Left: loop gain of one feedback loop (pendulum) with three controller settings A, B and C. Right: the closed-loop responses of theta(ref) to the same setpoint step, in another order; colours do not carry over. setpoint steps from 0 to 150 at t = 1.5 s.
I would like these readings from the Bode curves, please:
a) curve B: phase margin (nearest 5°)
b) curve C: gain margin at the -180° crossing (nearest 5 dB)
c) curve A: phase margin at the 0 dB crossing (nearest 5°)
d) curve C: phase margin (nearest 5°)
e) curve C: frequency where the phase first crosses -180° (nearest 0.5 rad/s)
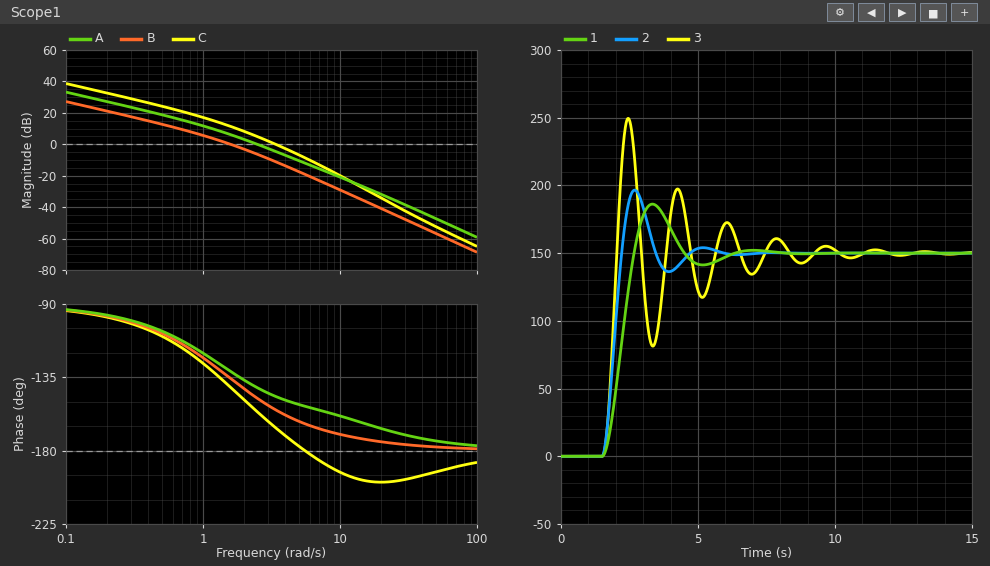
45°
10 dB
40°
15°
5.5 rad/s
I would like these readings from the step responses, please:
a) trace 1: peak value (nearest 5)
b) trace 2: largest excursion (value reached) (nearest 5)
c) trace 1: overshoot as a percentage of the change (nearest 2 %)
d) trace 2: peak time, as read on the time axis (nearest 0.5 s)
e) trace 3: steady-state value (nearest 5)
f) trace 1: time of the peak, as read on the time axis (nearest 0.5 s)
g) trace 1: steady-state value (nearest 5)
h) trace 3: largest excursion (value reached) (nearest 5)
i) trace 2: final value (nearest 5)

185
195
24 %
2.5 s
150
3.5 s
150
250
150
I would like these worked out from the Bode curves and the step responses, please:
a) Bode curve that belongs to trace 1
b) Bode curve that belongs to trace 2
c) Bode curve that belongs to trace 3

B
A
C
